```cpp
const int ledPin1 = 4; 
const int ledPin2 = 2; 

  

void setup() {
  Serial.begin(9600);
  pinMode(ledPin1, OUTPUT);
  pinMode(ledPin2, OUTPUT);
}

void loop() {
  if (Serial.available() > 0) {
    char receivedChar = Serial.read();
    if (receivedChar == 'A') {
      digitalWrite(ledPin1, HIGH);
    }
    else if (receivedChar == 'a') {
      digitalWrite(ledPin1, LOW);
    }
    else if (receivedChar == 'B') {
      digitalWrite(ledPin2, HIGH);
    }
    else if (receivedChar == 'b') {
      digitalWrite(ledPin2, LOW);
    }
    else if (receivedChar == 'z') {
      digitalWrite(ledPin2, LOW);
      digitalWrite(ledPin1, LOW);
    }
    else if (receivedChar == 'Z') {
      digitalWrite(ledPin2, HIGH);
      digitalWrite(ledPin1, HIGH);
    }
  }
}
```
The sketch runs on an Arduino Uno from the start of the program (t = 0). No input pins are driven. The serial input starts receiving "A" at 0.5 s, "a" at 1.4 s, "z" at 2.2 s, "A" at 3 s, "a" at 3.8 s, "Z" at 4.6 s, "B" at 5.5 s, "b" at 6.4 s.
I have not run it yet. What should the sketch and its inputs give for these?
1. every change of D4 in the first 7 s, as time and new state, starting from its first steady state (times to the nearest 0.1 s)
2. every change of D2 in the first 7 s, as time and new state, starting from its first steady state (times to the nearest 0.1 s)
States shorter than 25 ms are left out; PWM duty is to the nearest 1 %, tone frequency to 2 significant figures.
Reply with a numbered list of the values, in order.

1. 0 s low; 0.5 s high; 1.4 s low; 3 s high; 3.8 s low; 4.6 s high
2. 0 s low; 4.6 s high; 6.4 s low
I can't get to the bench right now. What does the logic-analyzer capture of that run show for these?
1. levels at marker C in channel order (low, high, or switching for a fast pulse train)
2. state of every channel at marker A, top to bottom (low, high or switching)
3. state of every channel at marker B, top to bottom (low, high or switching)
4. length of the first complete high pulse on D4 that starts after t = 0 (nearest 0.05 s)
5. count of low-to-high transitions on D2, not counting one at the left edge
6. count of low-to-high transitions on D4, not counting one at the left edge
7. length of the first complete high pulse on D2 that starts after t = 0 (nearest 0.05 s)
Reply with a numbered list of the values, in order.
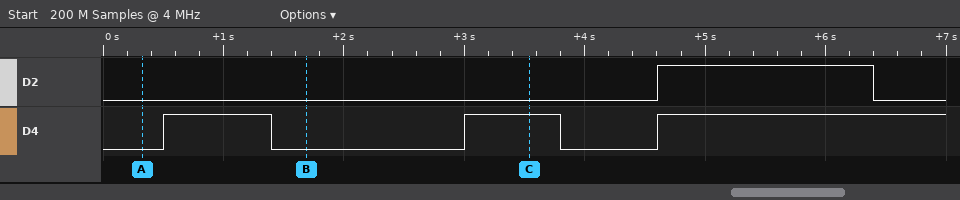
1. D2 low, D4 high
2. D2 low, D4 low
3. D2 low, D4 low
4. 0.90 s
5. 1
6. 3
7. 1.80 s
